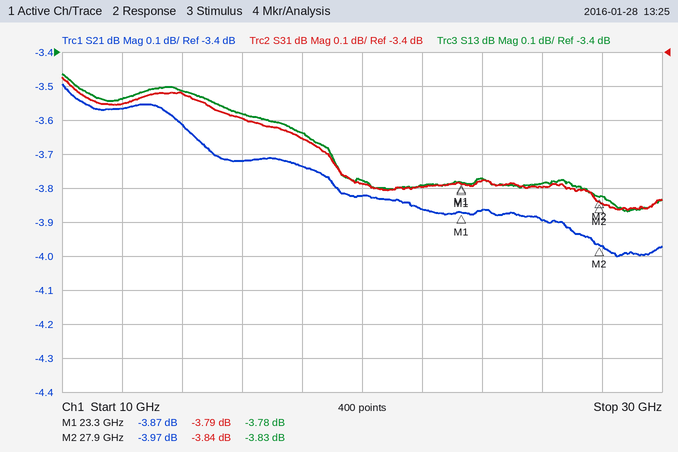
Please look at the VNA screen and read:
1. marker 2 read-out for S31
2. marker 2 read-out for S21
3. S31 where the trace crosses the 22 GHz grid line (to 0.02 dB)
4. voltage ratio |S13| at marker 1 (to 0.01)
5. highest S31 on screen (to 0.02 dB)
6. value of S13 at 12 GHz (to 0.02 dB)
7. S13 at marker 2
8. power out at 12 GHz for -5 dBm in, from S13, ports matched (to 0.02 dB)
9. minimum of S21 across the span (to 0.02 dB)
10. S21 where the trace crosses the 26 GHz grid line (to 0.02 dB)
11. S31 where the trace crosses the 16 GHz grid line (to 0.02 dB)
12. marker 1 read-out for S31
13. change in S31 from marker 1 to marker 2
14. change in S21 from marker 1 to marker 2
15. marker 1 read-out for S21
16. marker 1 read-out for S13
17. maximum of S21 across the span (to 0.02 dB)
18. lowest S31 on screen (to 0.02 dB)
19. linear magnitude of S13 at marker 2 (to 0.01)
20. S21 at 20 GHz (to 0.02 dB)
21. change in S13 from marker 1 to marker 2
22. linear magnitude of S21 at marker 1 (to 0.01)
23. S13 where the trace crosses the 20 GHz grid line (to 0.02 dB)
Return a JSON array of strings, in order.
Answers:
["-3.84 dB", "-3.97 dB", "-3.80 dB", "0.65", "-3.48 dB", "-3.54 dB", "-3.83 dB", "-8.54 dBm", "-4.00 dB", "-3.90 dB", "-3.60 dB", "-3.79 dB", "-0.05 dB", "-0.10 dB", "-3.87 dB", "-3.78 dB", "-3.50 dB", "-3.86 dB", "0.64", "-3.82 dB", "-0.05 dB", "0.64", "-3.78 dB"]
